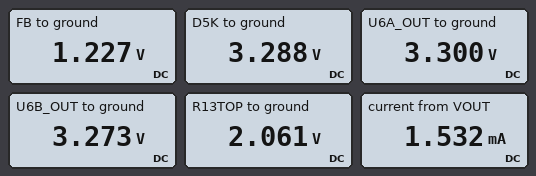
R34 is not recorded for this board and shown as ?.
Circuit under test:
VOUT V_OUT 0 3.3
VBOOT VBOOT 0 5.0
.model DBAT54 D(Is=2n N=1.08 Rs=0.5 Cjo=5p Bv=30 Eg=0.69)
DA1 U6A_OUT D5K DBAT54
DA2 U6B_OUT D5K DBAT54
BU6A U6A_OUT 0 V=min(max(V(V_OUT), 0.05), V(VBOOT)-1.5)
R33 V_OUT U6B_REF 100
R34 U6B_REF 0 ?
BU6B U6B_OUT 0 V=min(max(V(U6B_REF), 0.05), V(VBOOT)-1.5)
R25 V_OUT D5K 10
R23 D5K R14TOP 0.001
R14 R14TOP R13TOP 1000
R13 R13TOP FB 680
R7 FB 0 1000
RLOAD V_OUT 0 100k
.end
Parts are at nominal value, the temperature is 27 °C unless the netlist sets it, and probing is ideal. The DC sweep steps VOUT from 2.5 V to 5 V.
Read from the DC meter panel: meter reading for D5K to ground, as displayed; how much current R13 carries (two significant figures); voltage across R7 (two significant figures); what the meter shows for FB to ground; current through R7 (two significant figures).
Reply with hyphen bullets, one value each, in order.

- 3.288 V
- 1.2 mA
- 1.2 V
- 1.227 V
- 1.2 mA
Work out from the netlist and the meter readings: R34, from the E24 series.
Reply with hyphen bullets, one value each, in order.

- 12 kΩ
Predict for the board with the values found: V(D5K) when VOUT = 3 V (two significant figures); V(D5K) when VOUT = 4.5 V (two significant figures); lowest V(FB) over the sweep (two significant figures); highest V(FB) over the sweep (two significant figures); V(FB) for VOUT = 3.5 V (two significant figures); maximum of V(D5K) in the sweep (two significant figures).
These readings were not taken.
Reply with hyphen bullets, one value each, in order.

- 3.0 V
- 4.5 V
- 930 mV
- 1.9 V
- 1.3 V
- 5.0 V
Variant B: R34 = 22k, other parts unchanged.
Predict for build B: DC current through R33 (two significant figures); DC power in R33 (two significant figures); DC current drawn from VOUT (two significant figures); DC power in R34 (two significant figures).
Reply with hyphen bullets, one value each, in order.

- 150 µA
- 2.2 µW
- 1.4 mA
- 490 µW
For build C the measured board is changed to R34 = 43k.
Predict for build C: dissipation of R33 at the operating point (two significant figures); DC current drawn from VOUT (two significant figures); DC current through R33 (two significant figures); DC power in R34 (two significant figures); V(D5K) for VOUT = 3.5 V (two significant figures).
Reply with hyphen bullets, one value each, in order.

- 590 nW
- 1.3 mA
- 77 µA
- 250 µW
- 3.5 V
